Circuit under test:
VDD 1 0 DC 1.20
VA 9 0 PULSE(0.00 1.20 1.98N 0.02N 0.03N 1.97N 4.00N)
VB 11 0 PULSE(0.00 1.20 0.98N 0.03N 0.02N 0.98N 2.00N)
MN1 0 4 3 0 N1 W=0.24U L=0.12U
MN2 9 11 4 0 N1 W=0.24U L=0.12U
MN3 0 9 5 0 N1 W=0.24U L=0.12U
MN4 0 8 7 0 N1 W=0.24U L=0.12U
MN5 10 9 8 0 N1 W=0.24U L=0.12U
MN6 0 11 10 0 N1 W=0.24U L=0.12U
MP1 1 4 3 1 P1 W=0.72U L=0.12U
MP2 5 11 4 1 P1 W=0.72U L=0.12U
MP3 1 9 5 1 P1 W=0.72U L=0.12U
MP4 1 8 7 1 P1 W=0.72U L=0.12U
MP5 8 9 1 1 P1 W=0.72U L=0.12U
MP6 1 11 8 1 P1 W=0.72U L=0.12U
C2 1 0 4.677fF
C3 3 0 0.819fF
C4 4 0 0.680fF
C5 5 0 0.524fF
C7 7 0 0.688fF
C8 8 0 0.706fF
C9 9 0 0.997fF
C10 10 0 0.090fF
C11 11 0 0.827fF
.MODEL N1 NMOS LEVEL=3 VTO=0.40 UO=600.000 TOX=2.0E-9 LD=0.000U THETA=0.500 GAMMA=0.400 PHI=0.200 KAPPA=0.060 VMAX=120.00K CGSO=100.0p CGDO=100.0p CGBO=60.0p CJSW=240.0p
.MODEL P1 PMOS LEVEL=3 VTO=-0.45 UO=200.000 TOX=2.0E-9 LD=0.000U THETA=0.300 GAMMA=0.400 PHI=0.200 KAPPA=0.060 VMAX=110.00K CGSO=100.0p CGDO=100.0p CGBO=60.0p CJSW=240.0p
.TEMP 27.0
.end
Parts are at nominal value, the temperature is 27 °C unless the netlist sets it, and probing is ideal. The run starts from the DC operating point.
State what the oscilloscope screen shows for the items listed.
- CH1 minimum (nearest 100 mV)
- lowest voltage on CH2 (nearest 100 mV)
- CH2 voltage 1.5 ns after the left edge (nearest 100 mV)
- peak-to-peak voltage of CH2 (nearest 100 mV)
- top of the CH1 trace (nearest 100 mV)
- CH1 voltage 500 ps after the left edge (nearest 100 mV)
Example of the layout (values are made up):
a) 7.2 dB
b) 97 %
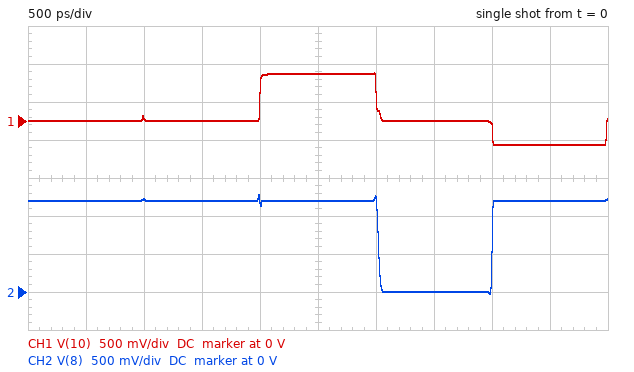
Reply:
a) -300 mV
b) 0 V
c) 1.2 V
d) 1.3 V
e) 600 mV
f) 0 V
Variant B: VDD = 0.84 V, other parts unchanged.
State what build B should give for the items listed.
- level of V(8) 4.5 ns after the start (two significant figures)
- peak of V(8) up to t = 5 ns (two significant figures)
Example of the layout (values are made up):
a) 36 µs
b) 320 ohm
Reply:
a) 840 mV
b) 960 mV
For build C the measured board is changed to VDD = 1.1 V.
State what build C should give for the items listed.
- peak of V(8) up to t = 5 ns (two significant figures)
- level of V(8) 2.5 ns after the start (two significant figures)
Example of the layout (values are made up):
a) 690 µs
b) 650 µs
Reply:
a) 1.2 V
b) 1.1 V
